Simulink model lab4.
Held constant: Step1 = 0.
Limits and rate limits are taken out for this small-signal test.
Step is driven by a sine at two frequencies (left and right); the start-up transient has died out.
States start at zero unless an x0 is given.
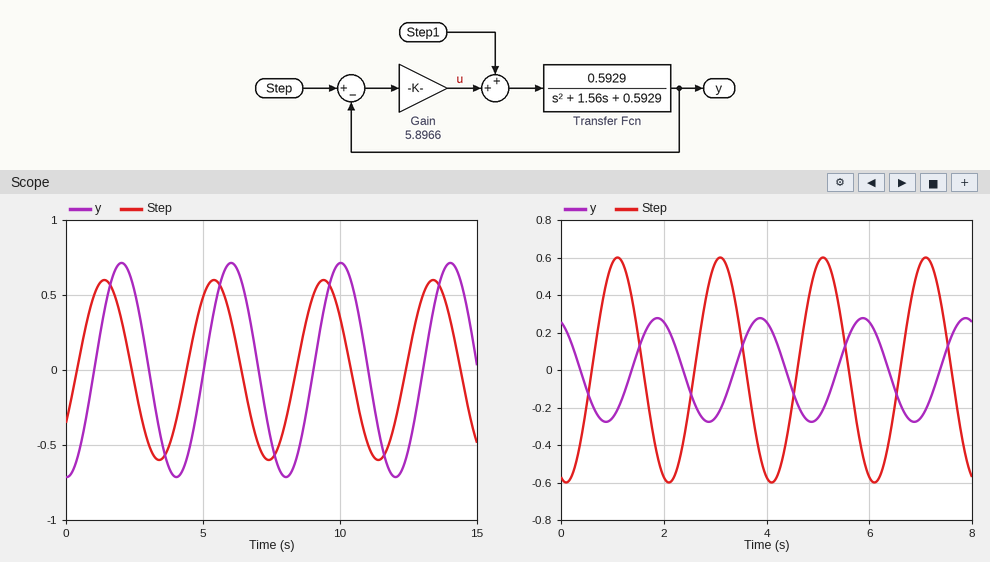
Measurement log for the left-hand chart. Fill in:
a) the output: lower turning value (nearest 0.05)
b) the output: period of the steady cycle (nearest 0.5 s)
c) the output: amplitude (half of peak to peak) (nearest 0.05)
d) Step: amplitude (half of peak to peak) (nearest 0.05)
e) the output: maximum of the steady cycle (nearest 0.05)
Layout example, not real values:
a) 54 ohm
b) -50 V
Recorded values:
a) -0.70
b) 4.0 s
c) 0.70
d) 0.60
e) 0.70
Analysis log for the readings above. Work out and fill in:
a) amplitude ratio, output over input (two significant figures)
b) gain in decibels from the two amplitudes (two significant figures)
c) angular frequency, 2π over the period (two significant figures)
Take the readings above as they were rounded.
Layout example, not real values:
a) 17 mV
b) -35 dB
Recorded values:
a) 1.2
b) 1.3 dB
c) 1.6 rad/s
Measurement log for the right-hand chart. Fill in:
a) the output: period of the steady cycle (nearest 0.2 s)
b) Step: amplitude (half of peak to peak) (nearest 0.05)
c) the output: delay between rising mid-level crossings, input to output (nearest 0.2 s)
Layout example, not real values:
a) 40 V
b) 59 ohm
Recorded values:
a) 2.0 s
b) 0.60
c) 0.8 s
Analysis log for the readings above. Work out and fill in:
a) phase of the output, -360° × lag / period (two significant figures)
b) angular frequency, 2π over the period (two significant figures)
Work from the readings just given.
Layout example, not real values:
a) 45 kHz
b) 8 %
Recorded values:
a) -140°
b) 3.1 rad/s
